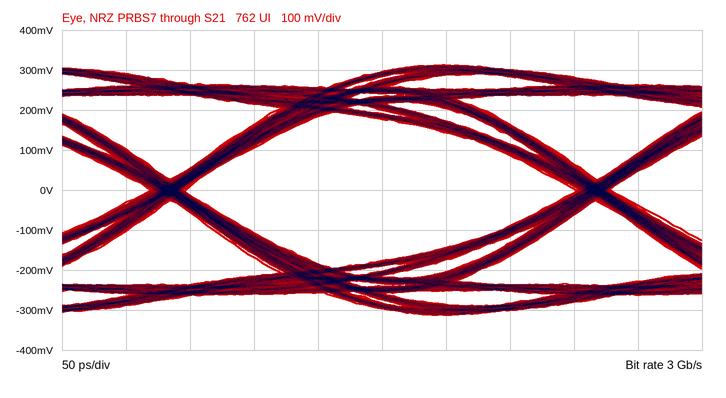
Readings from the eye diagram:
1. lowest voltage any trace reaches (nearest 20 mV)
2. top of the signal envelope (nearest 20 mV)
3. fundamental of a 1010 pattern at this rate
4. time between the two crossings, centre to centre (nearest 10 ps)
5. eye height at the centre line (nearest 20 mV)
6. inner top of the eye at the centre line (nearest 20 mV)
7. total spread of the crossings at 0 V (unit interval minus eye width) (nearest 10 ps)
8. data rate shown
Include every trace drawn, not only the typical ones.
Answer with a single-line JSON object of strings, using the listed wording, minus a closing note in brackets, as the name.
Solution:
{"lowest voltage any trace reaches": "-320 mV", "top of the signal envelope": "320 mV", "fundamental of a 1010 pattern at this rate": "1.5 GHz", "time between the two crossings, centre to centre": "330 ps", "eye height at the centre line": "360 mV", "inner top of the eye at the centre line": "180 mV", "total spread of the crossings at 0 V (unit interval minus eye width)": "30 ps", "data rate shown": "3 Gb/s"}
